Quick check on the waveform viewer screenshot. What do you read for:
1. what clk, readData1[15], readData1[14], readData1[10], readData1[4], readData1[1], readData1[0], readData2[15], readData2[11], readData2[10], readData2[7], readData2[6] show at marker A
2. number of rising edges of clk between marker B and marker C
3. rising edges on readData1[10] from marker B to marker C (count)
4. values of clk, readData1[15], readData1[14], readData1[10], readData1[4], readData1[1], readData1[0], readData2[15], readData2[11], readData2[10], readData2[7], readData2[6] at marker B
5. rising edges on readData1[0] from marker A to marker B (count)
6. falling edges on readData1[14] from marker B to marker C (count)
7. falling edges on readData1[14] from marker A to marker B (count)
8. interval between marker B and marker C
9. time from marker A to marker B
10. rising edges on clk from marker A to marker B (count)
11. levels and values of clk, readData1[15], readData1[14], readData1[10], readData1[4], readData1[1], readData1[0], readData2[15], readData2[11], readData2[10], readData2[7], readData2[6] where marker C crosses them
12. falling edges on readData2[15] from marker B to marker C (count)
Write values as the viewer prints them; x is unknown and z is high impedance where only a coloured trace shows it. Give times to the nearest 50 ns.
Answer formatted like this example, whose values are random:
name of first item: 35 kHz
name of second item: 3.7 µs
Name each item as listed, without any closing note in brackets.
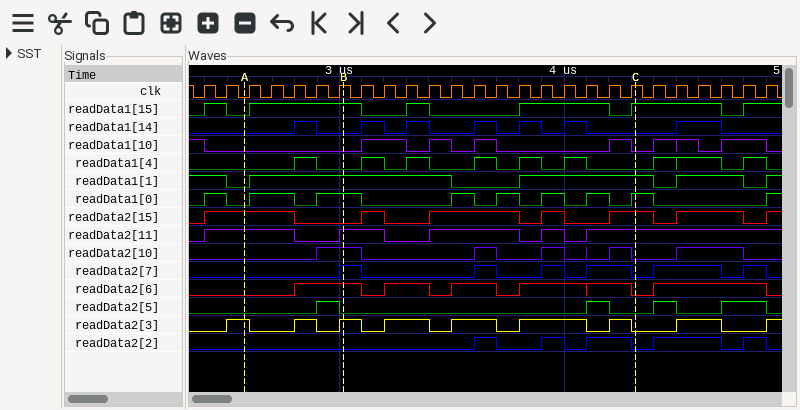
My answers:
what clk, readData1[15], readData1[14], readData1[10], readData1[4], readData1[1], readData1[0], readData2[15], readData2[11], readData2[10], readData2[7], readData2[6] show at marker A: clk=0, readData1[15]=0, readData1[14]=0, readData1[10]=0, readData1[4]=0, readData1[1]=0, readData1[0]=0, readData2[15]=1, readData2[11]=1, readData2[10]=0, readData2[7]=0, readData2[6]=0
number of rising edges of clk between marker B and marker C: 13
rising edges on readData1[10] from marker B to marker C: 4
values of clk, readData1[15], readData1[14], readData1[10], readData1[4], readData1[1], readData1[0], readData2[15], readData2[11], readData2[10], readData2[7], readData2[6] at marker B: clk=1, readData1[15]=1, readData1[14]=0, readData1[10]=0, readData1[4]=0, readData1[1]=1, readData1[0]=1, readData2[15]=0, readData2[11]=1, readData2[10]=1, readData2[7]=1, readData2[6]=1
rising edges on readData1[0] from marker A to marker B: 2
falling edges on readData1[14] from marker B to marker C: 5
falling edges on readData1[14] from marker A to marker B: 1
interval between marker B and marker C: 1300 ns
time from marker A to marker B: 450 ns
rising edges on clk from marker A to marker B: 5
levels and values of clk, readData1[15], readData1[14], readData1[10], readData1[4], readData1[1], readData1[0], readData2[15], readData2[11], readData2[10], readData2[7], readData2[6] where marker C crosses them: clk=1, readData1[15]=1, readData1[14]=0, readData1[10]=0, readData1[4]=0, readData1[1]=1, readData1[0]=1, readData2[15]=1, readData2[11]=1, readData2[10]=0, readData2[7]=0, readData2[6]=0
falling edges on readData2[15] from marker B to marker C: 3
